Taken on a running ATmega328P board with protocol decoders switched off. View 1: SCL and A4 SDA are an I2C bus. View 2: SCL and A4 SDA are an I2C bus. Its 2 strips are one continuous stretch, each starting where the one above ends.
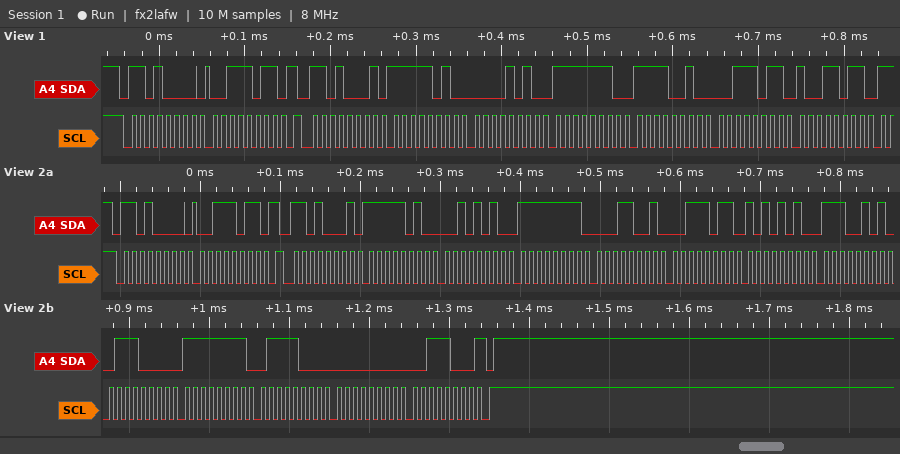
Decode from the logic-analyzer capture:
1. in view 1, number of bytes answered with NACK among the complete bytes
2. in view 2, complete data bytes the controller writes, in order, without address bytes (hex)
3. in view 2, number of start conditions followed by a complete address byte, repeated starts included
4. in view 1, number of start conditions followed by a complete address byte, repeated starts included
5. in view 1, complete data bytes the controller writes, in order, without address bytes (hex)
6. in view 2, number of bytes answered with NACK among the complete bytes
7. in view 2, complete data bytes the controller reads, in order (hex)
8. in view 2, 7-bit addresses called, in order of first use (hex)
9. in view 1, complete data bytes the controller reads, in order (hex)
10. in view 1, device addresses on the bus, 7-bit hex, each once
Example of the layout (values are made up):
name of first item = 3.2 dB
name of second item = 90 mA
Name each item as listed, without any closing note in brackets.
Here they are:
in view 1, number of bytes answered with NACK among the complete bytes = 0
in view 2, complete data bytes the controller writes, in order, without address bytes = 3B
in view 2, number of start conditions followed by a complete address byte, repeated starts included = 2
in view 1, number of start conditions followed by a complete address byte, repeated starts included = 2
in view 1, complete data bytes the controller writes, in order, without address bytes = 3B
in view 2, number of bytes answered with NACK among the complete bytes = 1
in view 2, complete data bytes the controller reads, in order = FA 2A FF 19 3B AA E5 70 FF 78 00 38
in view 2, 7-bit addresses called, in order of first use = 0x68
in view 1, complete data bytes the controller reads, in order = FA 0A FE F2 3B 9B
in view 1, device addresses on the bus, 7-bit hex, each once = 0x68
